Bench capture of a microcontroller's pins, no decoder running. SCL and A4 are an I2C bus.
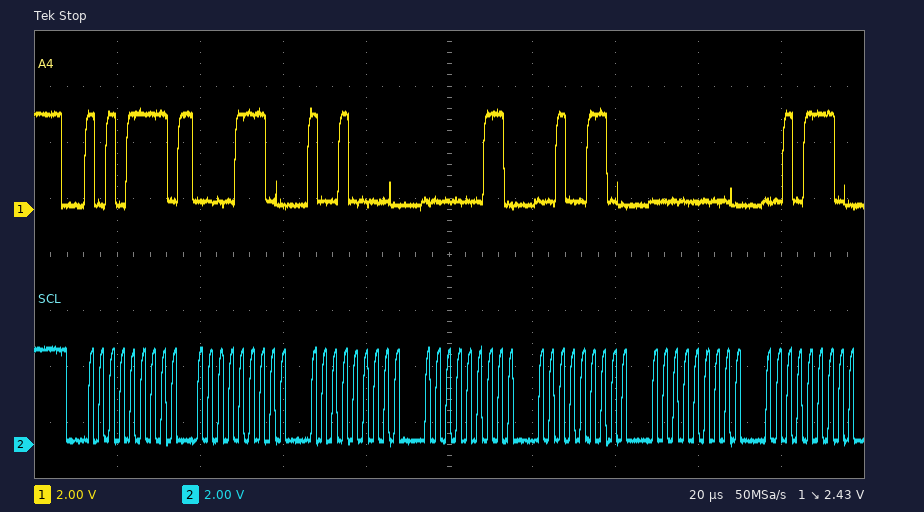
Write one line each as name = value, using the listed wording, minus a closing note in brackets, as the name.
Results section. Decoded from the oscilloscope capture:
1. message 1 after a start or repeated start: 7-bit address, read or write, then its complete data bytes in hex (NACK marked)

message 1 after a start or repeated start: 7-bit address, read or write, then its complete data bytes in hex = 0x57 read: 0E 90 03 26 00 2E
